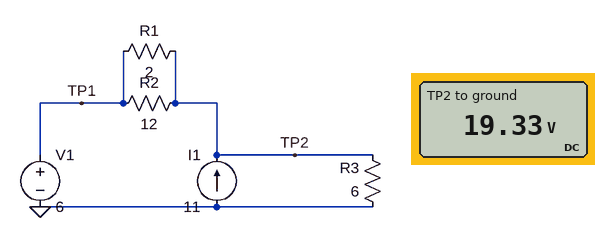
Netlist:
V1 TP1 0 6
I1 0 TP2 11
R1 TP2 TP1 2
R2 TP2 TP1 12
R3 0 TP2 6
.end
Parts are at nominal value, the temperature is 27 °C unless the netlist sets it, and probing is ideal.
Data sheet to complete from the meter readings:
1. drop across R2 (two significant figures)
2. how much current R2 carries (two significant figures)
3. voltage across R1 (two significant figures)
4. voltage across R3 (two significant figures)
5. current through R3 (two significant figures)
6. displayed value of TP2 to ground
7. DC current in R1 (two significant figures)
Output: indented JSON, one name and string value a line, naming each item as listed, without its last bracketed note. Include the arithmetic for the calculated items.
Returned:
{
  "drop across R2": "19.33 V - 6 V = 13 V",
  "how much current R2 carries": "(19.33 V - 6 V) / 12 Ω = 1.1 A",
  "voltage across R1": "19.33 V - 6 V = 13 V",
  "voltage across R3": "19.33 V = 19 V",
  "current through R3": "(19.33 V) / 6 Ω = 3.2 A",
  "displayed value of TP2 to ground": "19.33 V",
  "DC current in R1": "(19.33 V - 6 V) / 2 Ω = 6.7 A"
}
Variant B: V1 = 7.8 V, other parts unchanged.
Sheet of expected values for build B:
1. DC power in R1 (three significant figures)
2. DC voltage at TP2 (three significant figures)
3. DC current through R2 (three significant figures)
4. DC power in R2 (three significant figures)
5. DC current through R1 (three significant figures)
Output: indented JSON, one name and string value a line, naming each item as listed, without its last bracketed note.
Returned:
{
  "DC power in R1": "83.6 W",
  "DC voltage at TP2": "20.7 V",
  "DC current through R2": "1.08 A",
  "DC power in R2": "13.9 W",
  "DC current through R1": "6.47 A"
}
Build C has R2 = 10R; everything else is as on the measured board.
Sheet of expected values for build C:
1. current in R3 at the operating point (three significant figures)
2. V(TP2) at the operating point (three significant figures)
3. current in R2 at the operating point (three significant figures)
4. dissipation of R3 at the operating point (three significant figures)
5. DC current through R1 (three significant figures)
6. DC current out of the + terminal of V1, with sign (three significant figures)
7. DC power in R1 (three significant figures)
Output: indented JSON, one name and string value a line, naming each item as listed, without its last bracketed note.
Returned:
{
  "current in R3 at the operating point": "3.17 A",
  "V(TP2) at the operating point": "19.0 V",
  "current in R2 at the operating point": "1.30 A",
  "dissipation of R3 at the operating point": "60.4 W",
  "DC current through R1": "6.52 A",
  "DC current out of the + terminal of V1, with sign": "-7.83 A",
  "DC power in R1": "85.1 W"
}
